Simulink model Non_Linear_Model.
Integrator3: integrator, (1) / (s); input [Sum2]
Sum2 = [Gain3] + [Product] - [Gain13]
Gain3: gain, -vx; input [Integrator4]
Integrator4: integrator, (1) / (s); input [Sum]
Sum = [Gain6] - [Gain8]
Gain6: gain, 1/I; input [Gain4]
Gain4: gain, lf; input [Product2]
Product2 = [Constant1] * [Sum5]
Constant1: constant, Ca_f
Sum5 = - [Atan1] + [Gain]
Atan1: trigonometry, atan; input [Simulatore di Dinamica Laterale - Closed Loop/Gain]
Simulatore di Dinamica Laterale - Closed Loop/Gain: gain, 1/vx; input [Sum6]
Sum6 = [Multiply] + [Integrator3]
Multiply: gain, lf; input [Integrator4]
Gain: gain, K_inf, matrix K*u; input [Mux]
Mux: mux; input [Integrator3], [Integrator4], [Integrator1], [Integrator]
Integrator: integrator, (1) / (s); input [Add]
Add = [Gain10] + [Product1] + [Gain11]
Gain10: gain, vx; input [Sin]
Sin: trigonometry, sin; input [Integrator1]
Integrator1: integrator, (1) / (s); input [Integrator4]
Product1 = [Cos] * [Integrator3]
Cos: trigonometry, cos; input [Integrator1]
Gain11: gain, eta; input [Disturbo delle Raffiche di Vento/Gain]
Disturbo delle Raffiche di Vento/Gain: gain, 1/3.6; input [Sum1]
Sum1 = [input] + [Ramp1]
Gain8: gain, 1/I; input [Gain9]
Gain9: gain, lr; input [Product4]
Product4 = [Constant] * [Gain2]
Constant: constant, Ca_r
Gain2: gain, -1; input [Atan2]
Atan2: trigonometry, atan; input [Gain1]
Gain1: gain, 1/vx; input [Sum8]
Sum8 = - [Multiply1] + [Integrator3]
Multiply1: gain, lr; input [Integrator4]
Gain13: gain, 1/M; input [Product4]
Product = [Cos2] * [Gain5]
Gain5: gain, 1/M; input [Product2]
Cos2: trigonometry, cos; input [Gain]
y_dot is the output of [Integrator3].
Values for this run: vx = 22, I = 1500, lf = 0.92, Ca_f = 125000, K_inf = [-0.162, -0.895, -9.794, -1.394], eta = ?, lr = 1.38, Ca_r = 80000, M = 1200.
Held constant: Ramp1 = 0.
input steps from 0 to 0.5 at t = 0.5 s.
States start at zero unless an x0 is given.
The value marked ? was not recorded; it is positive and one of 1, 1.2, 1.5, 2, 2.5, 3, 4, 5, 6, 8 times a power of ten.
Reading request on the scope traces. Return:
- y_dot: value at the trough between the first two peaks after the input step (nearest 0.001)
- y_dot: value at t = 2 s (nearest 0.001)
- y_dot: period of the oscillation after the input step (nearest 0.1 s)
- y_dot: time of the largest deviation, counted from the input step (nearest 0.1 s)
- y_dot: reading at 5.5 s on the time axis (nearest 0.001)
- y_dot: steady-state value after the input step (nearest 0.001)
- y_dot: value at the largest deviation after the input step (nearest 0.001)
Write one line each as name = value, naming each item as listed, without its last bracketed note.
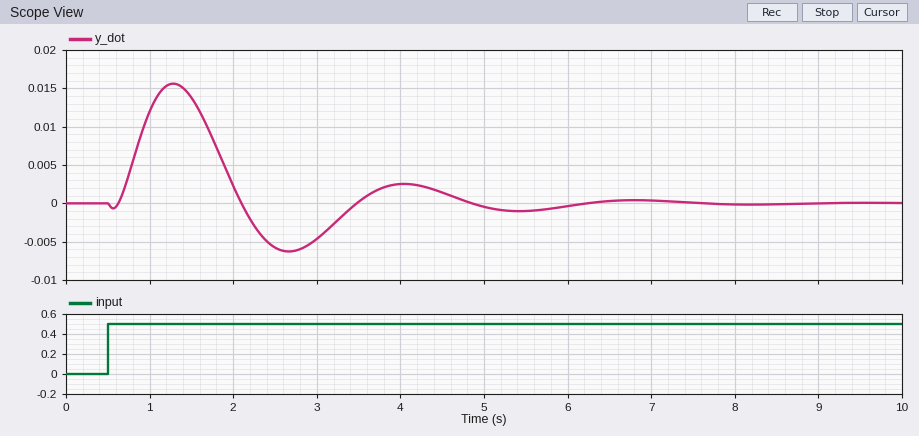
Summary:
y_dot: value at the trough between the first two peaks after the input step = -0.006
y_dot: value at t = 2 s = 0.002
y_dot: period of the oscillation after the input step = 2.8 s
y_dot: time of the largest deviation, counted from the input step = 0.8 s
y_dot: reading at 5.5 s on the time axis = -0.001
y_dot: steady-state value after the input step = 0.000
y_dot: value at the largest deviation after the input step = 0.016
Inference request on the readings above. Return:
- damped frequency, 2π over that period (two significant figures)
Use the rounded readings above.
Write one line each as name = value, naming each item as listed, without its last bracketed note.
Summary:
damped frequency, 2π over that period = 2.2 rad/s
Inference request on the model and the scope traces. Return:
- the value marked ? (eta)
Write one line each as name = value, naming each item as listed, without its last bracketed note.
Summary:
the value marked ? = 0.12
